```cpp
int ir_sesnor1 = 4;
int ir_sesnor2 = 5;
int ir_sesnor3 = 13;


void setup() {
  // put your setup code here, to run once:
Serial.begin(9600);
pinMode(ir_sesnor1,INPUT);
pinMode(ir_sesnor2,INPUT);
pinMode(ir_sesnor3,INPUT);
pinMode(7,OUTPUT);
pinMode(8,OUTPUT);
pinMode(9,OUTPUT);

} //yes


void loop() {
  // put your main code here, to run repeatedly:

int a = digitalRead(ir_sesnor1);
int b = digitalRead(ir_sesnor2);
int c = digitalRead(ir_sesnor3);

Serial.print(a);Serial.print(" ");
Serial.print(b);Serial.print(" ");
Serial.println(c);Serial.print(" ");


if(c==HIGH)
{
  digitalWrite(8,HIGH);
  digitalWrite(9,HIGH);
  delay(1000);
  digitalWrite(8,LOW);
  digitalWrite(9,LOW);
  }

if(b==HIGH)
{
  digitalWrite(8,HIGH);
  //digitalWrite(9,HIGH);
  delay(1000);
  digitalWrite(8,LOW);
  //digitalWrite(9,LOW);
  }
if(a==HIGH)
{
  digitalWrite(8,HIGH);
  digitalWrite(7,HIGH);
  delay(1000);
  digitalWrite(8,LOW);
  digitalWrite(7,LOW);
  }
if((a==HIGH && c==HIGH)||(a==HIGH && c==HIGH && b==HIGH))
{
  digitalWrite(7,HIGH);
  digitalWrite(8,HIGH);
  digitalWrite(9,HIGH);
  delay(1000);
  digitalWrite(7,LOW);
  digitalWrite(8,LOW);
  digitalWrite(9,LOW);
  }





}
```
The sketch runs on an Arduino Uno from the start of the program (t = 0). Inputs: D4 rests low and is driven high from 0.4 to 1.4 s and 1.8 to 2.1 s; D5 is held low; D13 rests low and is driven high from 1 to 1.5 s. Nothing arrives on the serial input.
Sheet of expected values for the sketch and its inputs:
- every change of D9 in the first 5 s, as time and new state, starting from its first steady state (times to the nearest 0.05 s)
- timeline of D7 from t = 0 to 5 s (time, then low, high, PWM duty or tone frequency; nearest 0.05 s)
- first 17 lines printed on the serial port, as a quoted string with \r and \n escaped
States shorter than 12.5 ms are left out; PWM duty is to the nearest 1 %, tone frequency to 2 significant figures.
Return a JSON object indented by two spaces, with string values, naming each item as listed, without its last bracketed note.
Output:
{
  "every change of D9 in the first 5 s, as time and new state, starting from its first steady state": "0 s low; 1.4 s high; 2.4 s low",
  "timeline of D7 from t = 0 to 5 s": "0 s low; 0.4 s high; 1.4 s low",
  "first 17 lines printed on the serial port, as a quoted string with \\r and \\n escaped": "\"0 0 0\\r\\n 0 0 0\\r\\n 0 0 0\\r\\n 0 0 0\\r\\n 0 0 0\\r\\n 0 0 0\\r\\n 0 0 0\\r\\n 0 0 0\\r\\n 0 0 0\\r\\n 0 0 0\\r\\n 0 0 0\\r\\n 0 0 0\\r\\n 0 0 0\\r\\n 0 0 0\\r\\n 0 0 0\\r\\n 0 0 0\\r\\n 0 0 0\\r\\n\""
}
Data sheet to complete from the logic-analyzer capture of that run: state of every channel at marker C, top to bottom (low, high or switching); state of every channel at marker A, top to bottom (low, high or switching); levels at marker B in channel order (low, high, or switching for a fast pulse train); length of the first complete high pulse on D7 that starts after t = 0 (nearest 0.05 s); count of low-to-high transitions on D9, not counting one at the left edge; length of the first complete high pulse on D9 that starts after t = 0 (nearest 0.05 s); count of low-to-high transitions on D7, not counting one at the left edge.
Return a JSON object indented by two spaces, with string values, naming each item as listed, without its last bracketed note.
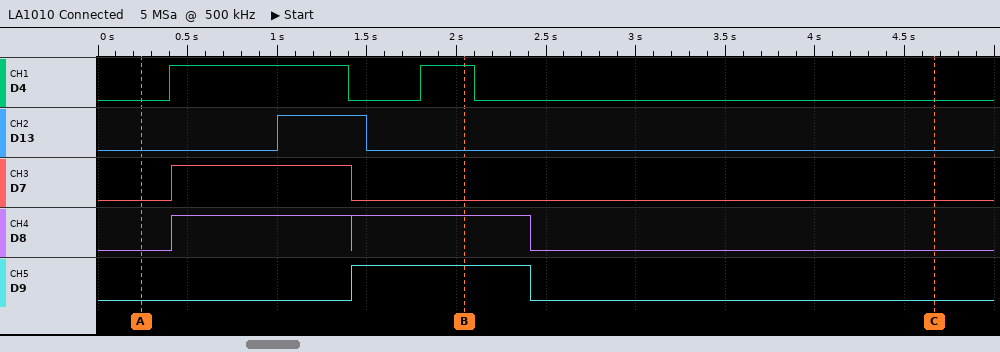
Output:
{
  "state of every channel at marker C, top to bottom": "D4 low, D13 low, D7 low, D8 low, D9 low",
  "state of every channel at marker A, top to bottom": "D4 low, D13 low, D7 low, D8 low, D9 low",
  "levels at marker B in channel order": "D4 high, D13 low, D7 low, D8 high, D9 high",
  "length of the first complete high pulse on D7 that starts after t = 0": "1.00 s",
  "count of low-to-high transitions on D9, not counting one at the left edge": "1",
  "length of the first complete high pulse on D9 that starts after t = 0": "1.00 s",
  "count of low-to-high transitions on D7, not counting one at the left edge": "1"
}
